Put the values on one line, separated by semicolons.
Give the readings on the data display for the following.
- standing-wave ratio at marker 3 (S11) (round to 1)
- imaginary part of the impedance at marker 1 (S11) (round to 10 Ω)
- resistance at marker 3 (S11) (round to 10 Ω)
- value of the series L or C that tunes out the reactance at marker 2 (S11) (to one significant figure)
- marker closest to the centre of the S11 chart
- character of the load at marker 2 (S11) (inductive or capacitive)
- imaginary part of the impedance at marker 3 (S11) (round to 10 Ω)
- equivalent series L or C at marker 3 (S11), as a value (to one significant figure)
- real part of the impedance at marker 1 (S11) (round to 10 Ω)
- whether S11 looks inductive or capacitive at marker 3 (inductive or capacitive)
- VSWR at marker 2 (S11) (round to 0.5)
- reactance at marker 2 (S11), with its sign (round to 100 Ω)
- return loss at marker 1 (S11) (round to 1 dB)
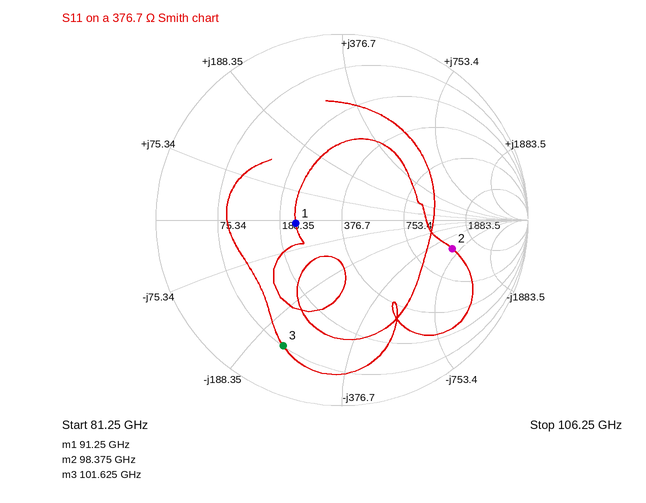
7; -10 Ω; 80 Ω; 1.0 nH; marker 1; capacitive; -230 Ω; 7 fF; 230 Ω; capacitive; 4.0; -600 Ω; 12 dB
